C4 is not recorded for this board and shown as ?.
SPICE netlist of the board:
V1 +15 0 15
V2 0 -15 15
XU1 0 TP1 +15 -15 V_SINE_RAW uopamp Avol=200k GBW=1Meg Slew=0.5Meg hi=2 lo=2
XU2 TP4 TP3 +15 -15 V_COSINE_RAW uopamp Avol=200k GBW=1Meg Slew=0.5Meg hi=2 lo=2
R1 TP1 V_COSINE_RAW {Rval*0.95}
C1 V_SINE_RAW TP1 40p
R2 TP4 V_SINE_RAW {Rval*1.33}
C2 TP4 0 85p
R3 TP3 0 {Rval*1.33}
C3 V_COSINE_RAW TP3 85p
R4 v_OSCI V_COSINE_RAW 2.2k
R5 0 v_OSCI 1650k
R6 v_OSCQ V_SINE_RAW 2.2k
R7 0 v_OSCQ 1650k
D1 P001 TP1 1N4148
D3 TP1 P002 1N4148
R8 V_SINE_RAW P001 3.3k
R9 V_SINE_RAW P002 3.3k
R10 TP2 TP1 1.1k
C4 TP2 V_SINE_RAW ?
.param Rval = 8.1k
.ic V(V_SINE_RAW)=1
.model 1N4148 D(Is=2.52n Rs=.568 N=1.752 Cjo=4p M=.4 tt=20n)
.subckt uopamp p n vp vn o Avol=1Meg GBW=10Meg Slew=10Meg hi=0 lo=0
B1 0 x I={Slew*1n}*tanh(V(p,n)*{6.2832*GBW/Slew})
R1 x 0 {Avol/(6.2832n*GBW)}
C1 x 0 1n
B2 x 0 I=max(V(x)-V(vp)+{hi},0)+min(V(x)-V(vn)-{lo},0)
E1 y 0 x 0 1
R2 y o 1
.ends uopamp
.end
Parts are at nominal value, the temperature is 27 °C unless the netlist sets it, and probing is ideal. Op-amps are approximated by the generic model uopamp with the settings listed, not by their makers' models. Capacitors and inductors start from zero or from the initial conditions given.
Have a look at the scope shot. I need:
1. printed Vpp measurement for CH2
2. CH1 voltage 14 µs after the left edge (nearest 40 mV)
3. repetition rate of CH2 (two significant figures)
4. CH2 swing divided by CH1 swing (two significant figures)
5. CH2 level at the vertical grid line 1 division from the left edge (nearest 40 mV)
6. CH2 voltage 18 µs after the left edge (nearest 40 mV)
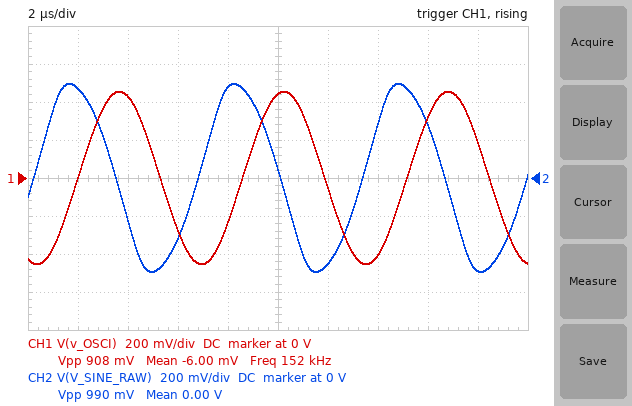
990 mV
-400 mV
150 kHz
1.1
480 mV
-480 mV
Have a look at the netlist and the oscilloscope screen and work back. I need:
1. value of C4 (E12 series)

33 pF
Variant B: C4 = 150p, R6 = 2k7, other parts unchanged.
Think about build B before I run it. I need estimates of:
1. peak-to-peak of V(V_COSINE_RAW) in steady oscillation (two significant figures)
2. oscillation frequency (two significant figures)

1.2 V
110 kHz
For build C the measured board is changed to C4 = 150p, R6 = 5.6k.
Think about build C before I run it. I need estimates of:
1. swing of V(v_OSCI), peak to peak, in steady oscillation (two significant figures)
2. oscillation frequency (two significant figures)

1.2 V
110 kHz
